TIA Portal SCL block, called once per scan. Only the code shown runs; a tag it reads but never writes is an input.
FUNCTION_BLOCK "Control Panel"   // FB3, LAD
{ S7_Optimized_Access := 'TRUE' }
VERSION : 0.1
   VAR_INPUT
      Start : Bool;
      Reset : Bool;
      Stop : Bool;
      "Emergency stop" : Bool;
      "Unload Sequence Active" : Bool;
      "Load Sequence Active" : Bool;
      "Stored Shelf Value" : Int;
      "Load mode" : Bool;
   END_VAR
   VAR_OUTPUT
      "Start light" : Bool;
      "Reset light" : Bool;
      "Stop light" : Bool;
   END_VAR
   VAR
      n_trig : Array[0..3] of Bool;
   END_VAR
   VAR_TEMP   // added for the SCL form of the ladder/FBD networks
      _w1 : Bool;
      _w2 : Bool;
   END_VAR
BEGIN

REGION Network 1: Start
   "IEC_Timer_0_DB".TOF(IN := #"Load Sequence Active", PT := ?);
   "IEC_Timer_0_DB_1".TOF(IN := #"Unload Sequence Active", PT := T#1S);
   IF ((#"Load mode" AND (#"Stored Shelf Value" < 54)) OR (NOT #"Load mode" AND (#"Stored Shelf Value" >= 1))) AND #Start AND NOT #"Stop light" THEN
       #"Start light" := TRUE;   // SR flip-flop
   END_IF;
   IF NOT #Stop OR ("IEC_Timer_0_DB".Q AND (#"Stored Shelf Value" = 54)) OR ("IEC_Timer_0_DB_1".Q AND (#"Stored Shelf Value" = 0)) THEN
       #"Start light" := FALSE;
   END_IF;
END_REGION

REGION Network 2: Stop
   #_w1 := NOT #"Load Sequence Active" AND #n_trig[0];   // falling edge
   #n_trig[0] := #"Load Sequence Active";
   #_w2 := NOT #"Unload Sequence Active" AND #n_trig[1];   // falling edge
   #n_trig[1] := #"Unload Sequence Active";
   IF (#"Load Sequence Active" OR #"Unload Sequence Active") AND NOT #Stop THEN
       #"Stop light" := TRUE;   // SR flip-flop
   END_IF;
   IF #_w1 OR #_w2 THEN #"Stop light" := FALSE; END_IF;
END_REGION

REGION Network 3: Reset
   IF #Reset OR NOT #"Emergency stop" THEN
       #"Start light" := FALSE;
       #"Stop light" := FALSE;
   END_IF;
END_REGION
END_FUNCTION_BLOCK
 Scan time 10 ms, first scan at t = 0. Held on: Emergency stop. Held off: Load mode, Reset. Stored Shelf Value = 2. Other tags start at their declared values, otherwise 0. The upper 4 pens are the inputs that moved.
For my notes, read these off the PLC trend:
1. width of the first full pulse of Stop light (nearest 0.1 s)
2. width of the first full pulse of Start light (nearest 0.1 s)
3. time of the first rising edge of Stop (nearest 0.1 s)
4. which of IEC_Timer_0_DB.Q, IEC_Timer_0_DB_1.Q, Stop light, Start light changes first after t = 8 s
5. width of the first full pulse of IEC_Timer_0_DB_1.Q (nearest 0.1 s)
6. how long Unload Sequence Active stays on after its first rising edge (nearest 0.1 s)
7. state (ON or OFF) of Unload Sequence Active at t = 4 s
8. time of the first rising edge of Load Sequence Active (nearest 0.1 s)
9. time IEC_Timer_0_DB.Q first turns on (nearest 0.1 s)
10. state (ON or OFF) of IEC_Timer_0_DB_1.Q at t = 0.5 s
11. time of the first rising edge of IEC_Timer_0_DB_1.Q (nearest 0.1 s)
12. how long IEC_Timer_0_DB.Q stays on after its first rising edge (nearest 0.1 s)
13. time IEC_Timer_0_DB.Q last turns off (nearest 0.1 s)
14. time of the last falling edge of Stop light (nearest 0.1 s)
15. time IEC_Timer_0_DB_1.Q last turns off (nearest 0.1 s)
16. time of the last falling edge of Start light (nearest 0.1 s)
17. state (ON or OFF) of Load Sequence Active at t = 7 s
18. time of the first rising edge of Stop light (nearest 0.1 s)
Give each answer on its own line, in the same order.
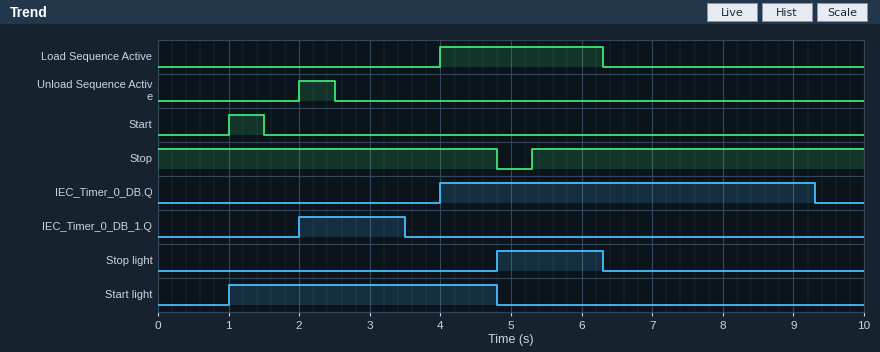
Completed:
1.5 s
3.8 s
5.3 s
IEC_Timer_0_DB.Q
1.5 s
0.5 s
OFF
4.0 s
4.0 s
OFF
2.0 s
5.3 s
9.3 s
6.3 s
3.5 s
4.8 s
OFF
4.8 s
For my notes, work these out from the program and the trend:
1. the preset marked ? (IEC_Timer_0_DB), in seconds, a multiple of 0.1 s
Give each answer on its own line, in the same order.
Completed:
3.0 s
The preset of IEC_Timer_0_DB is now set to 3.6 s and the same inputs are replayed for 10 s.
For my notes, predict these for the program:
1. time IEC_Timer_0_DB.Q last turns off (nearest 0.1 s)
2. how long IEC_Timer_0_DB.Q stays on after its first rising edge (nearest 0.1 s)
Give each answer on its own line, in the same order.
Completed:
9.9 s
5.9 s
